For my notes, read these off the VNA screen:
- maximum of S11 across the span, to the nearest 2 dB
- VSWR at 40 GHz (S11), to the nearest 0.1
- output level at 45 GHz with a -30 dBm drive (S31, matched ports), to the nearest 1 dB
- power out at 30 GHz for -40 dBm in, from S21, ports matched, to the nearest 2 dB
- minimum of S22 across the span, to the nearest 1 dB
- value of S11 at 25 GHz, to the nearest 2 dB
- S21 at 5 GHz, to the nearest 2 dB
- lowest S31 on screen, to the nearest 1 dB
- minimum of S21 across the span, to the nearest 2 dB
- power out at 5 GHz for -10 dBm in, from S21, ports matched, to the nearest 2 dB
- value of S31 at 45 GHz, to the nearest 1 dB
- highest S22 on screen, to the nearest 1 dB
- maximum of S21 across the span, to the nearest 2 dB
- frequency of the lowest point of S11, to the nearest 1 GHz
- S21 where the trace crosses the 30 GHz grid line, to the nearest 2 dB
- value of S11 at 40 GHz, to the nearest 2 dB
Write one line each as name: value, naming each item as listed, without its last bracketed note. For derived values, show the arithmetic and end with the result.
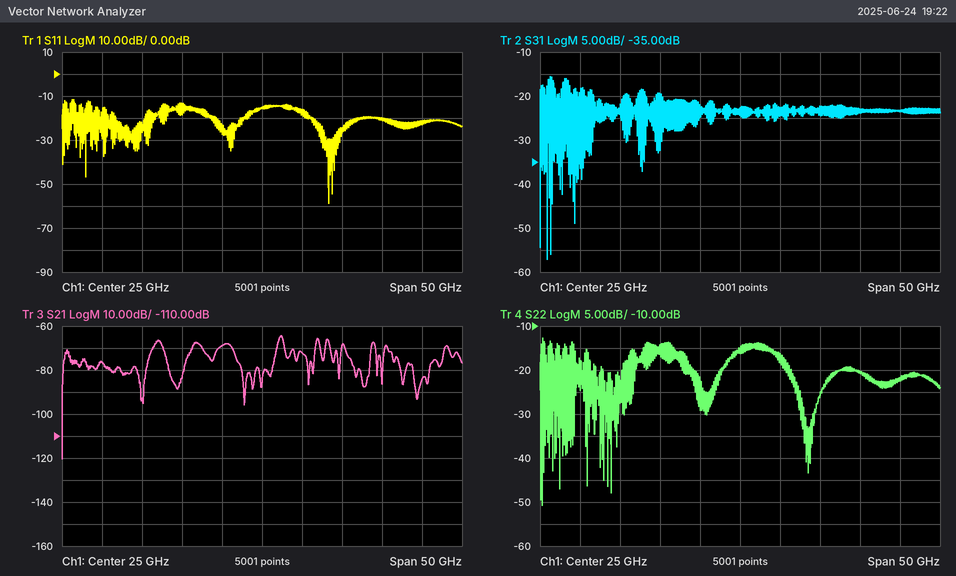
maximum of S11 across the span, to the nearest 2 dB: -12 dB
VSWR at 40 GHz (S11), to the nearest 0.1: |Γ| = 10^(-20/20) = 0.1000; VSWR = (1 + 0.1000)/(1 − 0.1000) ≈ 1.2
output level at 45 GHz with a -30 dBm drive (S31, matched ports), to the nearest 1 dB: -30 dBm + (-23 dB) = -53 dBm
power out at 30 GHz for -40 dBm in, from S21, ports matched, to the nearest 2 dB: -40 dBm + (-72 dB) = -112 dBm
minimum of S22 across the span, to the nearest 1 dB: -51 dB
value of S11 at 25 GHz, to the nearest 2 dB: -16 dB
S21 at 5 GHz, to the nearest 2 dB: -76 dB
lowest S31 on screen, to the nearest 1 dB: -57 dB
minimum of S21 across the span, to the nearest 2 dB: -120 dB
power out at 5 GHz for -10 dBm in, from S21, ports matched, to the nearest 2 dB: -10 dBm + (-76 dB) = -86 dBm
value of S31 at 45 GHz, to the nearest 1 dB: -23 dB
highest S22 on screen, to the nearest 1 dB: -13 dB
maximum of S21 across the span, to the nearest 2 dB: -64 dB
frequency of the lowest point of S11, to the nearest 1 GHz: 33 GHz
S21 where the trace crosses the 30 GHz grid line, to the nearest 2 dB: -72 dB
value of S11 at 40 GHz, to the nearest 2 dB: -20 dB
